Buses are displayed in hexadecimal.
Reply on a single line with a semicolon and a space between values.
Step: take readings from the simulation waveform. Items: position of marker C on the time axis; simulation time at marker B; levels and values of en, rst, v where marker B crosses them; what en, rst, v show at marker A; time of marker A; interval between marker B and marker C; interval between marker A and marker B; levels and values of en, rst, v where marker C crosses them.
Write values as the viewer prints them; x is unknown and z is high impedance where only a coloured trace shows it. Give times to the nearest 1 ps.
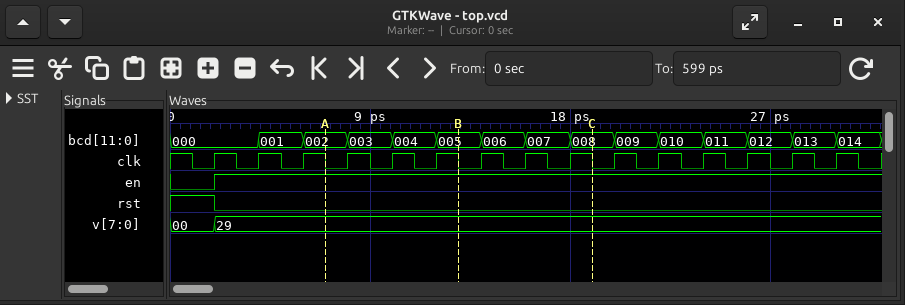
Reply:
19 ps; 13 ps; en=1, rst=0, v=29; en=1, rst=0, v=29; 7 ps; 6 ps; 6 ps; en=1, rst=0, v=29
